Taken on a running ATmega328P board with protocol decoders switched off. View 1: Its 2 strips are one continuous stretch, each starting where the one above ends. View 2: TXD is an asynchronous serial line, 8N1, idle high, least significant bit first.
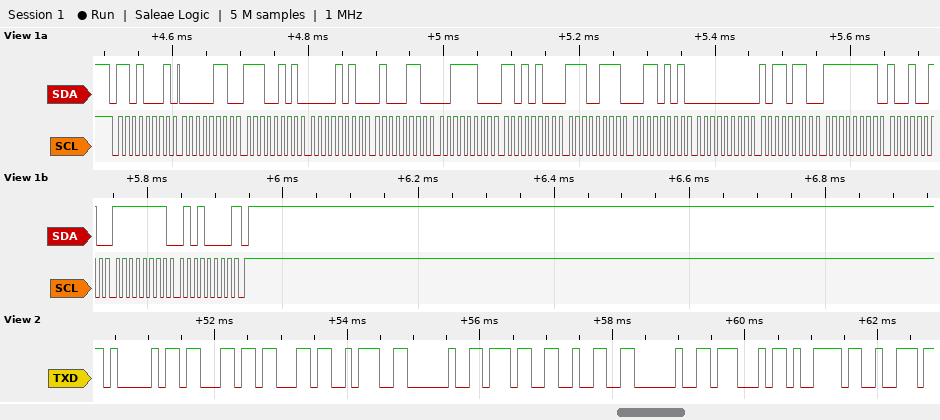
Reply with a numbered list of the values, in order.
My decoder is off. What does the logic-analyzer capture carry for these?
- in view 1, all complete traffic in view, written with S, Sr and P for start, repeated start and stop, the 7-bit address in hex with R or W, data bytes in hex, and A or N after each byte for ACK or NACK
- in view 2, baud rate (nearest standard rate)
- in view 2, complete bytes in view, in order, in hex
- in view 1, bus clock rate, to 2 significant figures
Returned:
1. S 68R A 06 A E5 A 0A A 46 A 3C A D4 A E7 A 35 A 00 A B6 A FF A 92 A FF A 50 N P
2. 9600 baud
3. 41 63 63 3A 20 37 32 20 47 79 72
4. 100 kHz
